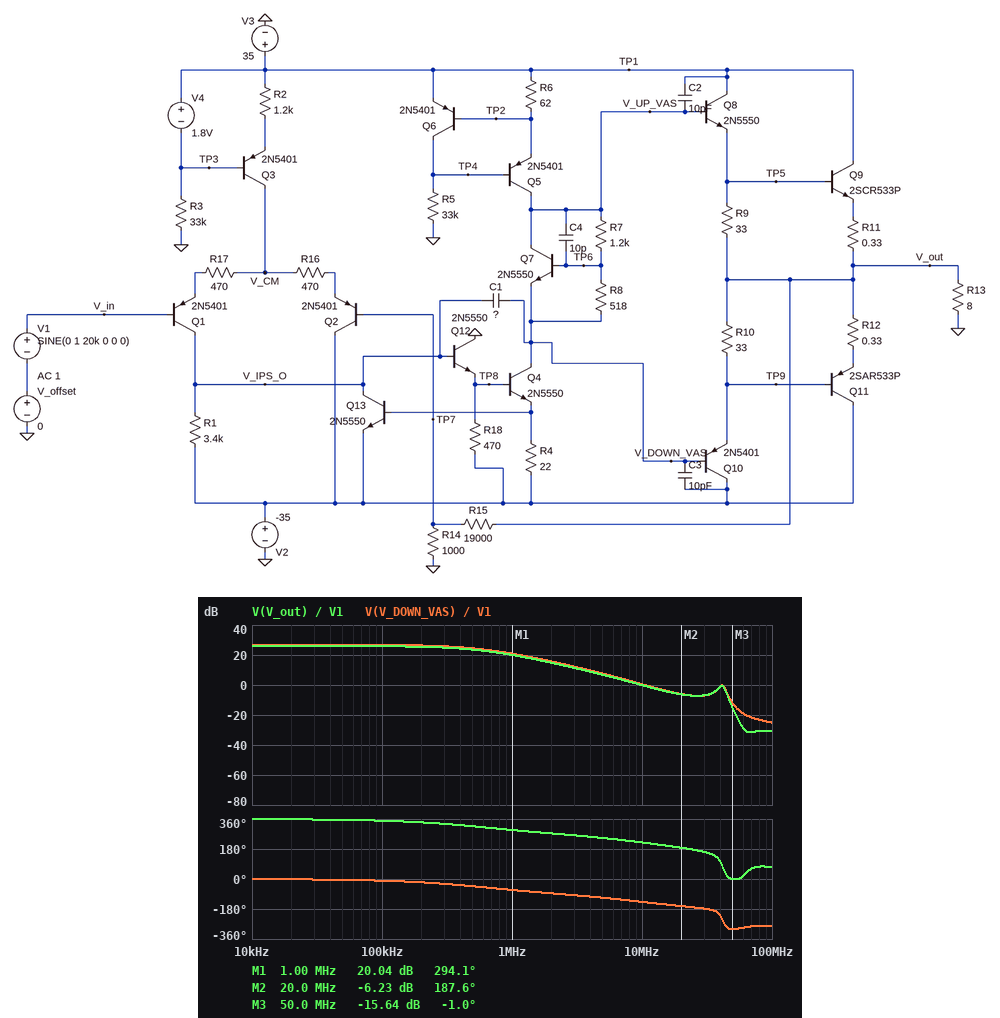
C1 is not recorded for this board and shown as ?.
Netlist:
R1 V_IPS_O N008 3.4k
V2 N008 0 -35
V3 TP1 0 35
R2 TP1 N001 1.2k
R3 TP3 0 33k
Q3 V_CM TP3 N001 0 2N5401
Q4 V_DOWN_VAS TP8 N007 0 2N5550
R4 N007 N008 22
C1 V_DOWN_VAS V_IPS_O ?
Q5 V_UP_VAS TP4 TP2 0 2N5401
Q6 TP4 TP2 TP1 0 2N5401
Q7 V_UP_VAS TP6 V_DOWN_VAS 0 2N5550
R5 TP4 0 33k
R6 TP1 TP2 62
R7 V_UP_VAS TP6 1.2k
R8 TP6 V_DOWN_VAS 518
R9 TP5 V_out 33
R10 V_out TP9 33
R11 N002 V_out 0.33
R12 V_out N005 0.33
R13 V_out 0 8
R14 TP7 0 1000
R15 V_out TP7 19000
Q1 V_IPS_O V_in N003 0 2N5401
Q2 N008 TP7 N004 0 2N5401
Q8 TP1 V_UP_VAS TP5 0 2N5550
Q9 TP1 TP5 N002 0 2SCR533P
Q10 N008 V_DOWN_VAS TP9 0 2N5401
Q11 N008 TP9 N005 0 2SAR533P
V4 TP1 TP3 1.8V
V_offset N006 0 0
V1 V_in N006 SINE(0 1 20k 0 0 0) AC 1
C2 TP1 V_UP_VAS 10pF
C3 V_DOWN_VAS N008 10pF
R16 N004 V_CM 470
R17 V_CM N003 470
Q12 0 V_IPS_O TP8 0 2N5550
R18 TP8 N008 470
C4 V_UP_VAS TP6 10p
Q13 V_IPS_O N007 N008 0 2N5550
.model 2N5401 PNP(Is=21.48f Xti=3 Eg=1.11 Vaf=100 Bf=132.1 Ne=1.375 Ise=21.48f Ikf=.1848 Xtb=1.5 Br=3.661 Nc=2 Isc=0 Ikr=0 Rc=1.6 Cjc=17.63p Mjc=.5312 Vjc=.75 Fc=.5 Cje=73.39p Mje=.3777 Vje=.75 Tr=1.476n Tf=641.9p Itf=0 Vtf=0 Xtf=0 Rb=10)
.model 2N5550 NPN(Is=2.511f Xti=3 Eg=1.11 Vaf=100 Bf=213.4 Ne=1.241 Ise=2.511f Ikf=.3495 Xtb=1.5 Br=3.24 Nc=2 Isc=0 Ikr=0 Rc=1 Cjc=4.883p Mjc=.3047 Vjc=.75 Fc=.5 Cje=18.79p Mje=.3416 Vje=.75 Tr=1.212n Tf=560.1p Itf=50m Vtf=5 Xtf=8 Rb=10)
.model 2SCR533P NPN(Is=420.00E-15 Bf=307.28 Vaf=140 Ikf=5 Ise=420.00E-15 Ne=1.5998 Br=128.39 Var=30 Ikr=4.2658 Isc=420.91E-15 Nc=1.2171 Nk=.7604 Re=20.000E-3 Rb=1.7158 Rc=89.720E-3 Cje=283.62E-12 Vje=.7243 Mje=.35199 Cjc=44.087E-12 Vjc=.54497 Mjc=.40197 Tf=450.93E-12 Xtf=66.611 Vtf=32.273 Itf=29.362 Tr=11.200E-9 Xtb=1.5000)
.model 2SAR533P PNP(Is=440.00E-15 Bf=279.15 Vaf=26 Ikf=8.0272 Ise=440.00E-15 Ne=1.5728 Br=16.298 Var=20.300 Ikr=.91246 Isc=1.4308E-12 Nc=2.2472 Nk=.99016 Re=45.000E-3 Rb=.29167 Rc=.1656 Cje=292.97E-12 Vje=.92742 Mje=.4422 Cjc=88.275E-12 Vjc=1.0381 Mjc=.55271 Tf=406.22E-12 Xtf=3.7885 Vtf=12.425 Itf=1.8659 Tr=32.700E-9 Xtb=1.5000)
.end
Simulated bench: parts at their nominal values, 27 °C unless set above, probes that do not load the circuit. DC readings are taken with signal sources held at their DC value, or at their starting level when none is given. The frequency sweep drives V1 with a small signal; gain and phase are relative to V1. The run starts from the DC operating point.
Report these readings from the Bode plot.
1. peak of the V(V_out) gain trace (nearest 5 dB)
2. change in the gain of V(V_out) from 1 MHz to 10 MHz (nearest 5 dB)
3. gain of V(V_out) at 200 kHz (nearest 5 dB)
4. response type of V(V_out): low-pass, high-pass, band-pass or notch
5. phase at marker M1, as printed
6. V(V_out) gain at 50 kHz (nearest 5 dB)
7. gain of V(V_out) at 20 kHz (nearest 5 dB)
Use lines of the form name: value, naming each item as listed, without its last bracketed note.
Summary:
peak of the V(V_out) gain trace: 25 dB
change in the gain of V(V_out) from 1 MHz to 10 MHz: -20 dB
gain of V(V_out) at 200 kHz: 25 dB
response type of V(V_out): low-pass, high-pass, band-pass or notch: low-pass
phase at marker M1, as printed: 294.1 deg
V(V_out) gain at 50 kHz: 25 dB
gain of V(V_out) at 20 kHz: 25 dB
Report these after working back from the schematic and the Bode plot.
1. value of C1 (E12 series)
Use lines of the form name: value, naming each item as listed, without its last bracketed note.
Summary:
value of C1: 12 pF
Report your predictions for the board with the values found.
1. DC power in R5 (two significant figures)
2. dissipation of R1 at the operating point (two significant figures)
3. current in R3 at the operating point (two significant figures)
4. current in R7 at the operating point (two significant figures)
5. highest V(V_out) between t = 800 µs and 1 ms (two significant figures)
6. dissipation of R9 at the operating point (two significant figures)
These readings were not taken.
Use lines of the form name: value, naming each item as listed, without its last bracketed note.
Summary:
DC power in R5: 34 mW
dissipation of R1 at the operating point: 820 µW
current in R3 at the operating point: 1.0 mA
current in R7 at the operating point: 1.5 mA
highest V(V_out) between t = 800 µs and 1 ms: 20 V
dissipation of R9 at the operating point: 14 mW
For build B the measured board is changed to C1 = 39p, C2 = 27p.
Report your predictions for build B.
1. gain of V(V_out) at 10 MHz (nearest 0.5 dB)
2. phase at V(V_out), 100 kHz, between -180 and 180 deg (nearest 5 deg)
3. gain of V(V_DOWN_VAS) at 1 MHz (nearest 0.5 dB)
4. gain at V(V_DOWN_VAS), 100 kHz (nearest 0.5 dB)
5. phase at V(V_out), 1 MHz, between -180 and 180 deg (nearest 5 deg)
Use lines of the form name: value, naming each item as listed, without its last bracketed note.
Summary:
gain of V(V_out) at 10 MHz: -10.5 dB
phase at V(V_out), 100 kHz, between -180 and 180 deg: -30 deg
gain of V(V_DOWN_VAS) at 1 MHz: 11.5 dB
gain at V(V_DOWN_VAS), 100 kHz: 25.5 dB
phase at V(V_out), 1 MHz, between -180 and 180 deg: -85 deg
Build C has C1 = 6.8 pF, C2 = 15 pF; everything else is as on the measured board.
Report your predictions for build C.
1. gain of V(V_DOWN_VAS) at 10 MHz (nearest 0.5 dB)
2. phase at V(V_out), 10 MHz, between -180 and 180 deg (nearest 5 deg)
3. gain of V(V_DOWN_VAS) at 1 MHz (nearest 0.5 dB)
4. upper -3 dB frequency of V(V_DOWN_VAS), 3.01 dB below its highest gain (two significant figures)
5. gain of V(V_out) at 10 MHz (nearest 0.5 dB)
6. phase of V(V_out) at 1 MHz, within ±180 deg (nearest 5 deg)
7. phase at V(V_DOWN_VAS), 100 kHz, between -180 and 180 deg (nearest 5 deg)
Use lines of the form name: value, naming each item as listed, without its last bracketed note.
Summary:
gain of V(V_DOWN_VAS) at 10 MHz: 5.5 dB
phase at V(V_out), 10 MHz, between -180 and 180 deg: -145 deg
gain of V(V_DOWN_VAS) at 1 MHz: 24.0 dB
upper -3 dB frequency of V(V_DOWN_VAS), 3.01 dB below its highest gain: 1.1 MHz
gain of V(V_out) at 10 MHz: 5.0 dB
phase of V(V_out) at 1 MHz, within ±180 deg: -50 deg
phase at V(V_DOWN_VAS), 100 kHz, between -180 and 180 deg: -5 deg
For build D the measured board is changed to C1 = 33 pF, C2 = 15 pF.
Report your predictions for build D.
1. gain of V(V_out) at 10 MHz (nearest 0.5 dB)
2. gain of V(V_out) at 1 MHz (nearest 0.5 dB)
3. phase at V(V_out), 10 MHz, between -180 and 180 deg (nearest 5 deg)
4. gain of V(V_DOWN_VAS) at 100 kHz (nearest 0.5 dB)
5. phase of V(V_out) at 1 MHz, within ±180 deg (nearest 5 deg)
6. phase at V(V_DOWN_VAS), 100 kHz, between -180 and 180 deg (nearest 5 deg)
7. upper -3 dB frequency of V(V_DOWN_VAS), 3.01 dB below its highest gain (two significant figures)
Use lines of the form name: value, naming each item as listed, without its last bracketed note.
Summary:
gain of V(V_out) at 10 MHz: -9.0 dB
gain of V(V_out) at 1 MHz: 12.0 dB
phase at V(V_out), 10 MHz, between -180 and 180 deg: -145 deg
gain of V(V_DOWN_VAS) at 100 kHz: 26.0 dB
phase of V(V_out) at 1 MHz, within ±180 deg: -85 deg
phase at V(V_DOWN_VAS), 100 kHz, between -180 and 180 deg: -25 deg
upper -3 dB frequency of V(V_DOWN_VAS), 3.01 dB below its highest gain: 210 kHz
